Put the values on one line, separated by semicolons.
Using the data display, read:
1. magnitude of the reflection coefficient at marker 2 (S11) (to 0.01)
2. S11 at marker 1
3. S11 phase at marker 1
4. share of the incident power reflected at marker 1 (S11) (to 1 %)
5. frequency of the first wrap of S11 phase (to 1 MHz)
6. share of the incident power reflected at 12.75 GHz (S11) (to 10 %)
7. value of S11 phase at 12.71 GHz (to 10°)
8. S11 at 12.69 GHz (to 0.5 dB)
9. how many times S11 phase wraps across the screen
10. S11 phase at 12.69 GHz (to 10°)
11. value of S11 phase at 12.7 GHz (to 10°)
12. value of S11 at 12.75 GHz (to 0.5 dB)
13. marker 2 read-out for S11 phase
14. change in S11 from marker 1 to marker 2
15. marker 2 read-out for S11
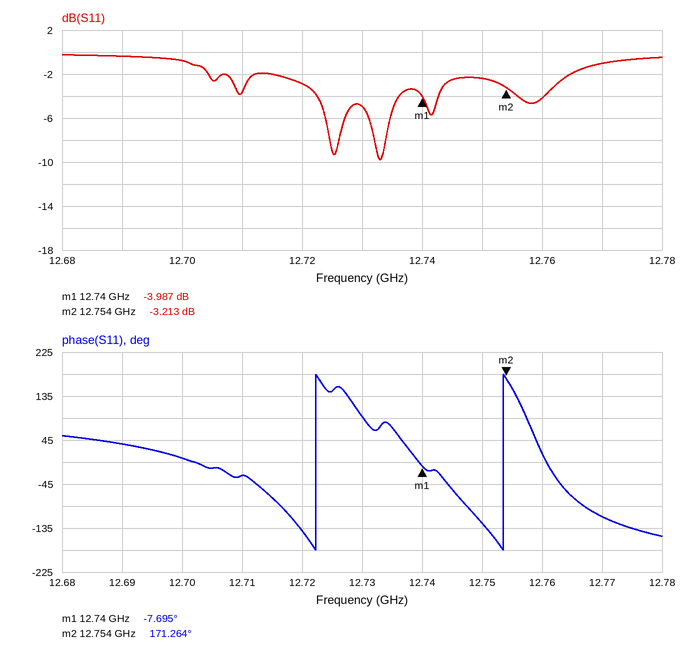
0.69; -3.987 dB; -7.695°; 40 %; 12.722 GHz; 60 %; -30°; -0.5 dB; 2; 40°; 10°; -2.5 dB; 171.264°; 0.774 dB; -3.213 dB
